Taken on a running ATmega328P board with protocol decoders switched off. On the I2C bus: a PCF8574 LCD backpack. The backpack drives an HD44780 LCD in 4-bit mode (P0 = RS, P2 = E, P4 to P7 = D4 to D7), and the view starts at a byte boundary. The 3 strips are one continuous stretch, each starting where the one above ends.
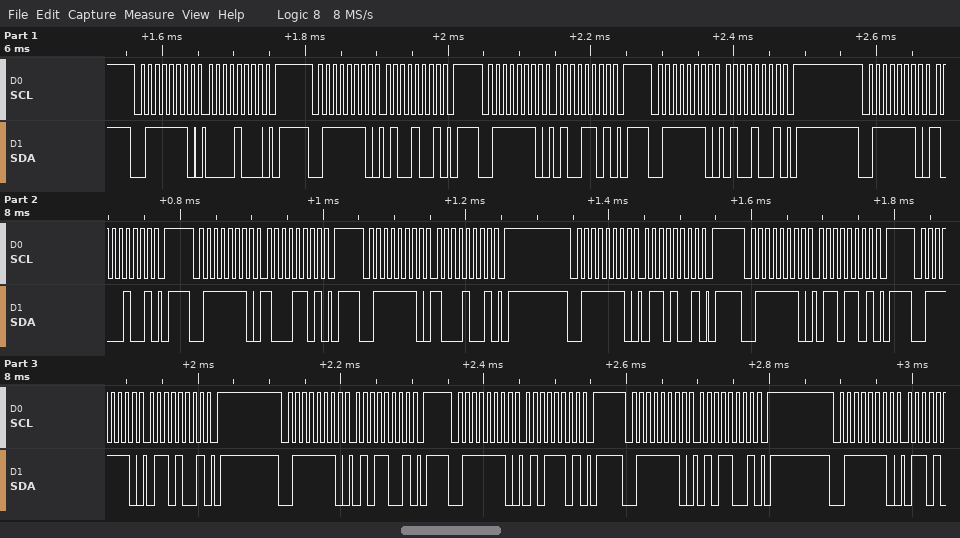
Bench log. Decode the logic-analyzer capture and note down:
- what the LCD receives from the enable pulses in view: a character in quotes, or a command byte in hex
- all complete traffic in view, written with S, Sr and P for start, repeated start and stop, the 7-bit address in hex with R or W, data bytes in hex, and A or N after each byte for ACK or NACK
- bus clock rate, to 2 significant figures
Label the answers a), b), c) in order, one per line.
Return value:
a) 'H' 'e'
b) S 3FW A 08 A P S 3FW A 49 A P S 3FW A 4D A P S 3FW A 49 A P S 3FW A 89 A P S 3FW A 8D A P S 3FW A 89 A P S 3FW A 69 A P S 3FW A 6D A P S 3FW A 69 A P S 3FW A 59 A P S 3FW A 5D A P S 3FW A 59 A P S 3FW A
c) 100 kHz
